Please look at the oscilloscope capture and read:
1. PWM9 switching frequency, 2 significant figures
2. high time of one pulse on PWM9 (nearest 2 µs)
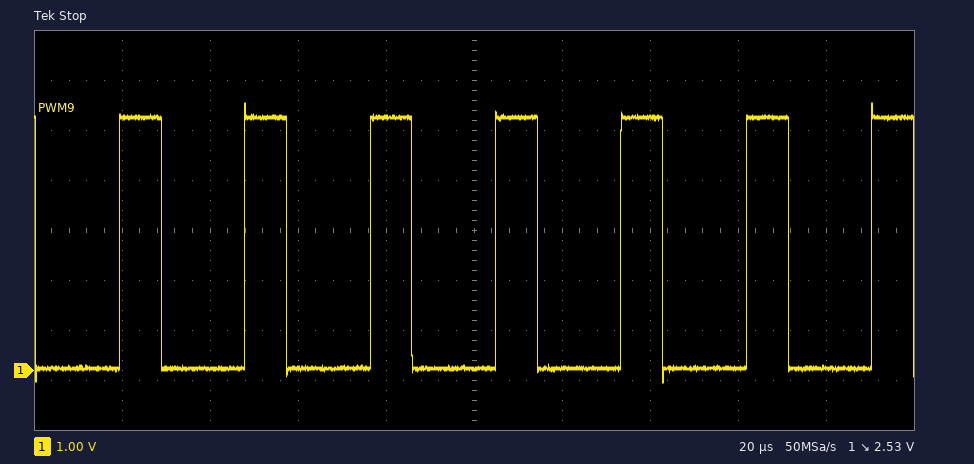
35 kHz
10 µs
